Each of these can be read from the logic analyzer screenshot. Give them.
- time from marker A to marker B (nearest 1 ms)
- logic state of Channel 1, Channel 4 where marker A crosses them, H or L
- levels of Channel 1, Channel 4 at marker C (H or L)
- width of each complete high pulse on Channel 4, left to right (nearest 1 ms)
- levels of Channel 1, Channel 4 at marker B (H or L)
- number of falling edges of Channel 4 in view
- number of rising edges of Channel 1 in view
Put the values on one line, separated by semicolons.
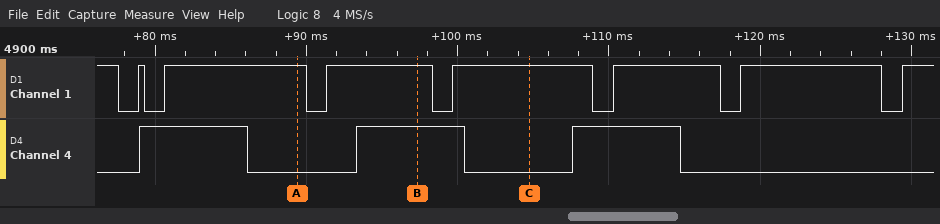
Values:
8 ms; Channel 1=H, Channel 4=L; Channel 1=H, Channel 4=L; 7 ms, 7 ms, 7 ms; Channel 1=H, Channel 4=H; 3; 7
